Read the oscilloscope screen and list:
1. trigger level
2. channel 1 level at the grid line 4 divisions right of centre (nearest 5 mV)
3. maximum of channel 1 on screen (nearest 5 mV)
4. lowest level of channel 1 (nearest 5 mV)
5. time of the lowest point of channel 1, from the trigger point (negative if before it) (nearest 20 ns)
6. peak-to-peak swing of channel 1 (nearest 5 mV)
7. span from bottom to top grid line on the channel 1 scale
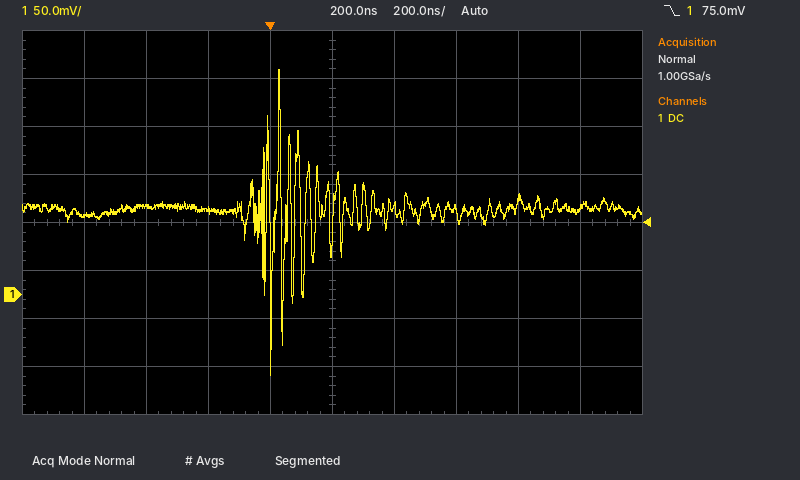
75.0 mV
90 mV
235 mV
-85 mV
0 ns
320 mV
400 mV
